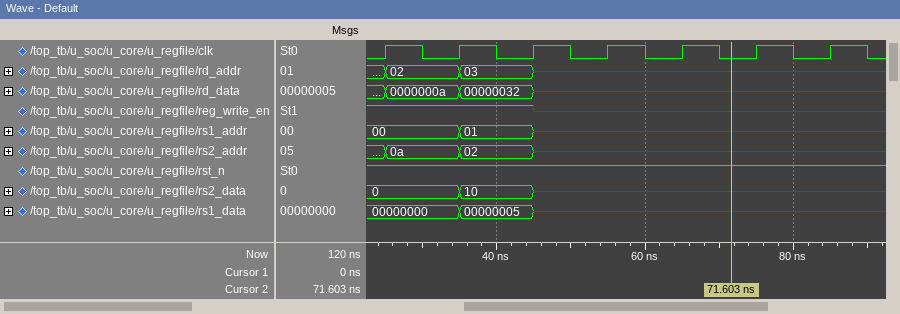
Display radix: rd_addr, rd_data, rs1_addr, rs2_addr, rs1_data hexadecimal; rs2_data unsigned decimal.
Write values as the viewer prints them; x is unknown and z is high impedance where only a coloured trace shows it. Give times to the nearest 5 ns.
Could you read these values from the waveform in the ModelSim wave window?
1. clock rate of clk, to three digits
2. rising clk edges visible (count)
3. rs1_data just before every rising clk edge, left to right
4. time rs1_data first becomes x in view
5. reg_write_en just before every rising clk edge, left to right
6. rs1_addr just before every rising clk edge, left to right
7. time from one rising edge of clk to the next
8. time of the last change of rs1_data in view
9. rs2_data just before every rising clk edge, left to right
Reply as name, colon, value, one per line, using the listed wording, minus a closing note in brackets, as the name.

clock rate of clk, to three digits: 100 MHz
rising clk edges visible: 7
rs1_data just before every rising clk edge, left to right: 00000000, 00000000, 00000005, x, x, x, x
time rs1_data first becomes x in view: 45 ns
reg_write_en just before every rising clk edge, left to right: 1 1 1 x x x x
rs1_addr just before every rising clk edge, left to right: 00, 00, 01, x, x, x, x
time from one rising edge of clk to the next: 10 ns
time of the last change of rs1_data in view: 45 ns
rs2_data just before every rising clk edge, left to right: 0, 0, 10, x, x, x, x
